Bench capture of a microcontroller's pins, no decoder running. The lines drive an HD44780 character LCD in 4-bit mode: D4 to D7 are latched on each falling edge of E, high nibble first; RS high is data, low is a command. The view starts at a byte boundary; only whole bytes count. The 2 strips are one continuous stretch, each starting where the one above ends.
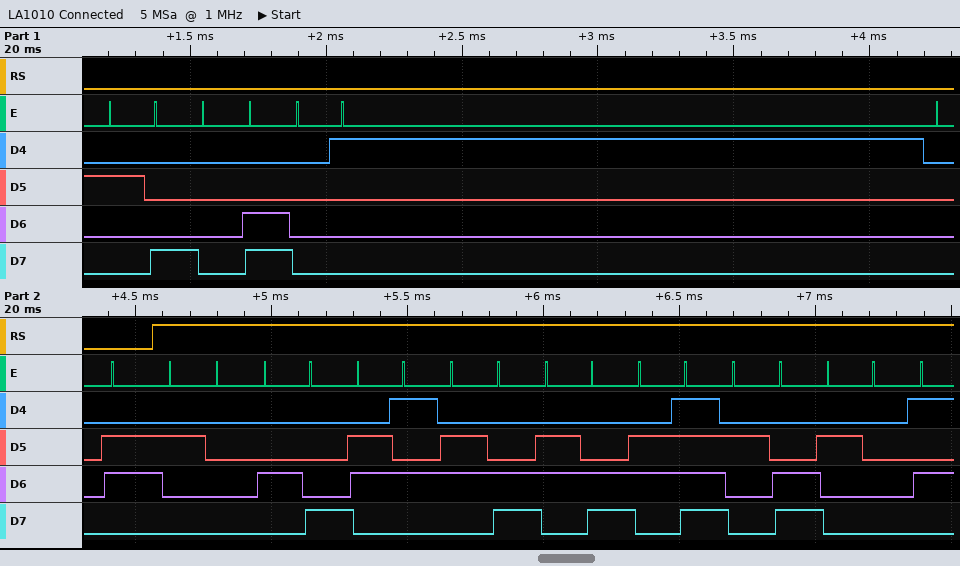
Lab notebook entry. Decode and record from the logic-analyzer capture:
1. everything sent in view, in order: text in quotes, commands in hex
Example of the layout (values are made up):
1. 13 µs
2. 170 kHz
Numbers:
1. 0x28 0x0C 0x01 0x06 " Hello, "
